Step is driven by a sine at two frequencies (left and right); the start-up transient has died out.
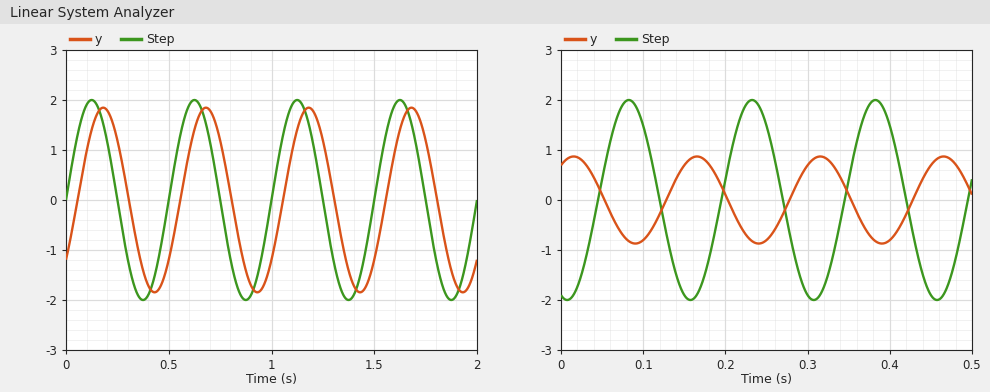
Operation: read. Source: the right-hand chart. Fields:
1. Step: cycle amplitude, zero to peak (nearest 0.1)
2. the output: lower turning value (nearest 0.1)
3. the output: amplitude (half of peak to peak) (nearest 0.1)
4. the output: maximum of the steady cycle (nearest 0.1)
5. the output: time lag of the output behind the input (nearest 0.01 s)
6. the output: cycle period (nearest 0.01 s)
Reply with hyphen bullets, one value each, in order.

- 2.0
- -0.9
- 0.9
- 0.9
- 0.08 s
- 0.15 s
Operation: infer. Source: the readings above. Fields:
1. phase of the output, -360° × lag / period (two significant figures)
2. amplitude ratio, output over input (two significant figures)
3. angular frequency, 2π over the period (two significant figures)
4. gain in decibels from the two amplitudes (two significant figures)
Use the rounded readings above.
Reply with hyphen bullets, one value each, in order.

- -190°
- 0.45
- 42 rad/s
- -6.9 dB
